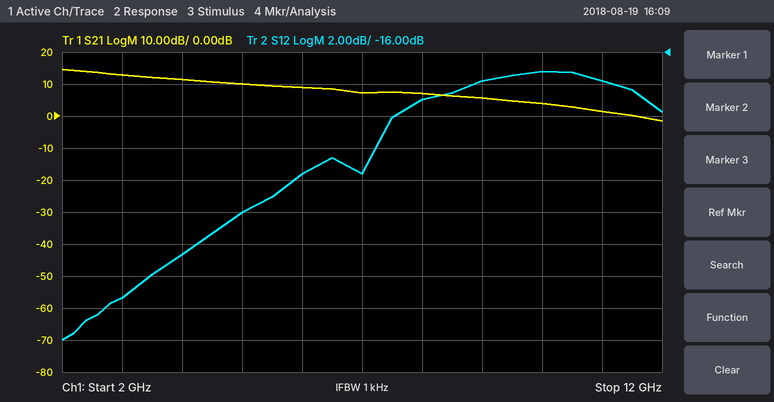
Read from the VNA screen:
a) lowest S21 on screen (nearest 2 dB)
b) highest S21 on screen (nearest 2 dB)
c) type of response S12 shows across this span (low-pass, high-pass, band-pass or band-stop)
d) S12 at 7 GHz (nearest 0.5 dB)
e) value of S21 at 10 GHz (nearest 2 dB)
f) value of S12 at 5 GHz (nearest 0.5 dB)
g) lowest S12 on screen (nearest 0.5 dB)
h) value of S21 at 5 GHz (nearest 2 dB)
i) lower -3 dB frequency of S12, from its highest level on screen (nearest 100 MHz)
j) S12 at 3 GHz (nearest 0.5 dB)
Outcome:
-2 dB
14 dB
high-pass
-23.5 dB
4 dB
-26.0 dB
-34.0 dB
10 dB
7.5 GHz
-31.5 dB
